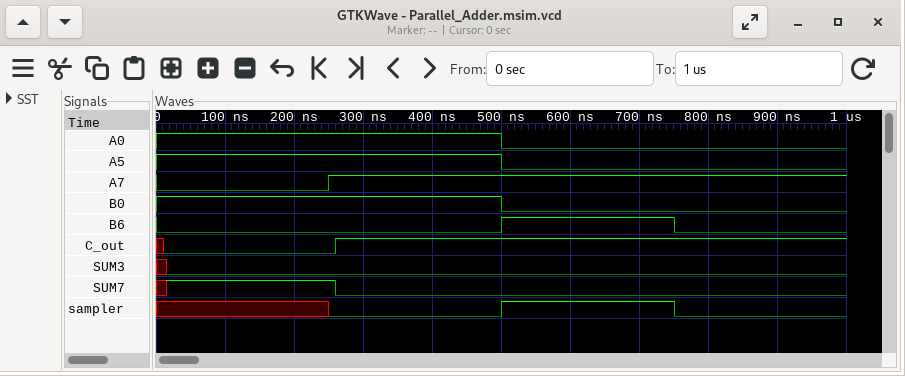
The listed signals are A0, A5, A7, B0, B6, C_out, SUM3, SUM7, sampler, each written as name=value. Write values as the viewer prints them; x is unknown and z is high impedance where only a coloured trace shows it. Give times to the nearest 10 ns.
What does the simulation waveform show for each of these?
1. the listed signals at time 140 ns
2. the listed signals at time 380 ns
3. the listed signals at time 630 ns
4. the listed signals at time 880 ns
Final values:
A0=1, A5=1, A7=0, B0=1, B6=0, C_out=0, SUM3=0, SUM7=1, sampler=x
A0=1, A5=1, A7=1, B0=1, B6=0, C_out=1, SUM3=0, SUM7=0, sampler=0
A0=0, A5=0, A7=1, B0=0, B6=1, C_out=1, SUM3=0, SUM7=0, sampler=1
A0=0, A5=0, A7=1, B0=0, B6=0, C_out=1, SUM3=0, SUM7=0, sampler=0
